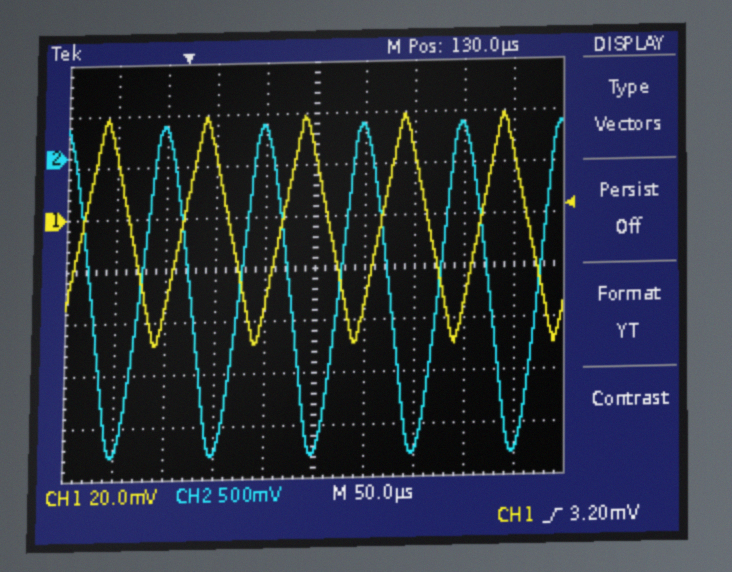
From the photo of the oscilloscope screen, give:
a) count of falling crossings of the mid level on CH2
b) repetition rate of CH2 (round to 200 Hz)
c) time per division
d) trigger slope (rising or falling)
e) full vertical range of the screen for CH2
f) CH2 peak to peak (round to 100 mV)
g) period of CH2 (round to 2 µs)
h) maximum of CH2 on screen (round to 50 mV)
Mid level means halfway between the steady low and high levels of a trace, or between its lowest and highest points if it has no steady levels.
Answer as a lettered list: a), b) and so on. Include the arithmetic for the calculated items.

a) 5
b) 1 / 100 µs ≈ 10.0 kHz
c) 50 µs
d) rising
e) 4 V
f) 3.20 V
g) 100 µs
h) 300 mV
